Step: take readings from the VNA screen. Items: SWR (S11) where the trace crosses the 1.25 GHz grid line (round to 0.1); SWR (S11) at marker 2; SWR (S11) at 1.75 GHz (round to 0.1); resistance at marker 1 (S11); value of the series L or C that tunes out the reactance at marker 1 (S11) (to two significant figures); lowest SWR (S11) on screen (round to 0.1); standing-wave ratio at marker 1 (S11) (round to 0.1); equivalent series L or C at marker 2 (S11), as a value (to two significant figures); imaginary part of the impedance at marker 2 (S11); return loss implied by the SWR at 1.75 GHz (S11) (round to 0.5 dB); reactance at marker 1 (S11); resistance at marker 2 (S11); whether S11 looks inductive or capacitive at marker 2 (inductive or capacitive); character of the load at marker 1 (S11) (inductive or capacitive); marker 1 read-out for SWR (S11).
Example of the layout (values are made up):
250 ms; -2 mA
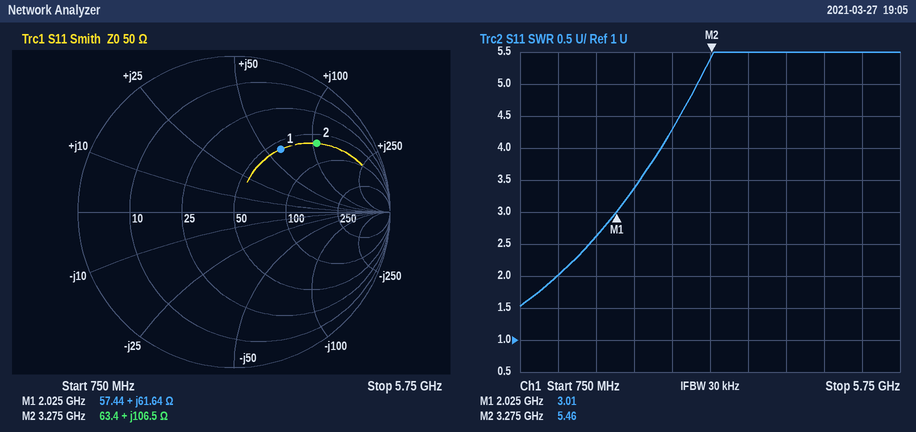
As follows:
2.0; 5.46; 2.6; 57.44 Ω; 1.3 pF; 1.5; 3.0; 5.2 nH; +106.5 Ω; 7.0 dB; +61.64 Ω; 63.4 Ω; inductive; inductive; 3.01
